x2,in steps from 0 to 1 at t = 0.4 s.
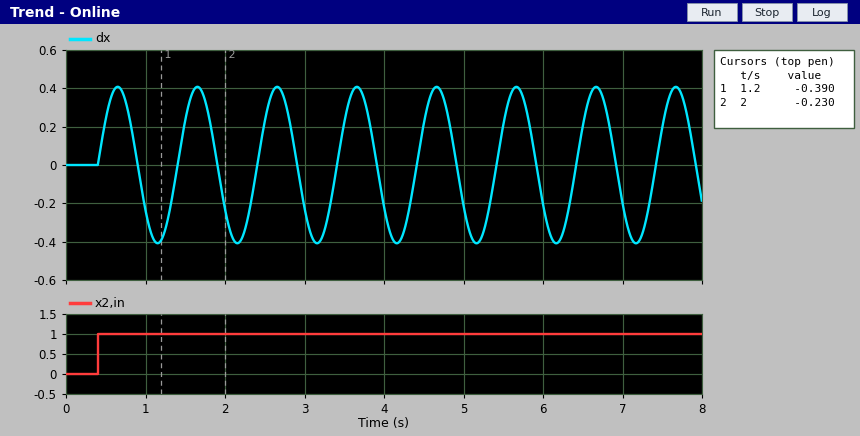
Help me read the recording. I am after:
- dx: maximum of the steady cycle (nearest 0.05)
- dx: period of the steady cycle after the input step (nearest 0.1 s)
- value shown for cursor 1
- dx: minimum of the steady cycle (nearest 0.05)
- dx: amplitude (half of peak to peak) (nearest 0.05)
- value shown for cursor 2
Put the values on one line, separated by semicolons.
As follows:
0.40; 1.0 s; -0.390; -0.40; 0.40; -0.230
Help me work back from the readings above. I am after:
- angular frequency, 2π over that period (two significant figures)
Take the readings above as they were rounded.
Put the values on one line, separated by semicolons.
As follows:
6.3 rad/s
